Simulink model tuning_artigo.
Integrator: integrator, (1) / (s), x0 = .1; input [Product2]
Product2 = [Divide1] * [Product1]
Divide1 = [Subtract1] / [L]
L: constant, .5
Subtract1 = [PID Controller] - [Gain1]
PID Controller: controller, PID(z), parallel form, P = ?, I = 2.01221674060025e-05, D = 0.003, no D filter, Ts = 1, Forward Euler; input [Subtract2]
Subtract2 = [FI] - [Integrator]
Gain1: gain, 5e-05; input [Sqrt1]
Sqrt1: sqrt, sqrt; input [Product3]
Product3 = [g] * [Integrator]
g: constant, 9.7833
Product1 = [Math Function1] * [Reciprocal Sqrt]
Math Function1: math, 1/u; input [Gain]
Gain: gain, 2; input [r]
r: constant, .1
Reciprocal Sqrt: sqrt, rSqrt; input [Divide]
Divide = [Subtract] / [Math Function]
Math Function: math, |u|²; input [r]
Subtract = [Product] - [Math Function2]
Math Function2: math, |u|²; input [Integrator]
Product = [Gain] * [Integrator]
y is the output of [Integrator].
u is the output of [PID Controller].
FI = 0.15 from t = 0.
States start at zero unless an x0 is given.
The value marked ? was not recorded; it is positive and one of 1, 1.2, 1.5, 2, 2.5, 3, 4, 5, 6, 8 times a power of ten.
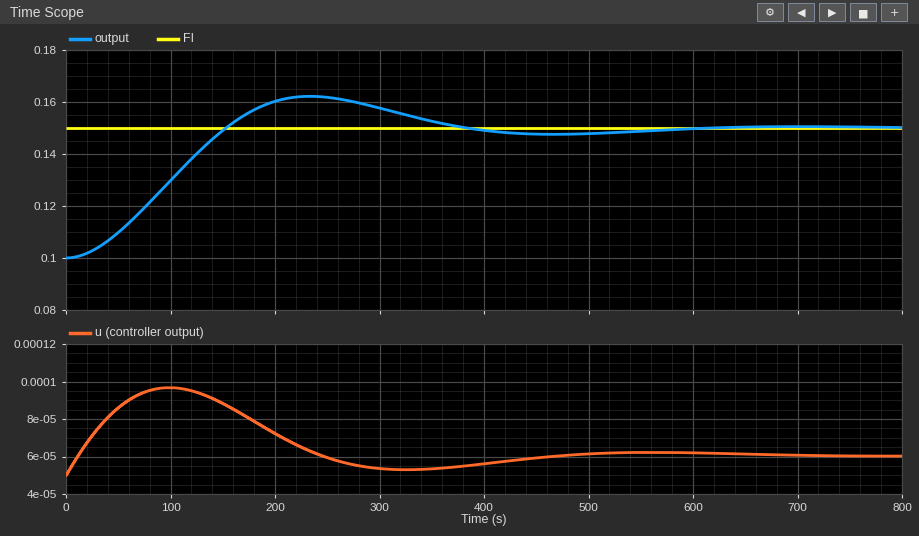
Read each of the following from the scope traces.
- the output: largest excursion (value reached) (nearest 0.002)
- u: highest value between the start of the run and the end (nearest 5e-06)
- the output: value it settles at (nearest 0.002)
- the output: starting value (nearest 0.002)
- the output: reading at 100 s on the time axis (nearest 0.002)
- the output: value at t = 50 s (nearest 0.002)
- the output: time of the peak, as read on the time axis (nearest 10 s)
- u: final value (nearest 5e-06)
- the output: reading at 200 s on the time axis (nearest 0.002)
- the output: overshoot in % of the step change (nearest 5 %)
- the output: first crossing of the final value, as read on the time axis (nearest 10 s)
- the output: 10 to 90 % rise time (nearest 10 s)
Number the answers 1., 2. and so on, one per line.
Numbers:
1. 0.162
2. 0.000095
3. 0.150
4. 0.100
5. 0.130
6. 0.110
7. 230 s
8. 0.000060
9. 0.160
10. 25 %
11. 150 s
12. 100 s
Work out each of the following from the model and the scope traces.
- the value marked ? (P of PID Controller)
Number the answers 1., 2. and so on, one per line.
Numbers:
1. 0.001
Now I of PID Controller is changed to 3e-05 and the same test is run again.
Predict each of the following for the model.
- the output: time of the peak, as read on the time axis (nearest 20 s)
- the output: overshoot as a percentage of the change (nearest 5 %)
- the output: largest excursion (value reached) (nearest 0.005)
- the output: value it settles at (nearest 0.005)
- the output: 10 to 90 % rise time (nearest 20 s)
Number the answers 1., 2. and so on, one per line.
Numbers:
1. 180 s
2. 35 %
3. 0.165
4. 0.150
5. 80 s
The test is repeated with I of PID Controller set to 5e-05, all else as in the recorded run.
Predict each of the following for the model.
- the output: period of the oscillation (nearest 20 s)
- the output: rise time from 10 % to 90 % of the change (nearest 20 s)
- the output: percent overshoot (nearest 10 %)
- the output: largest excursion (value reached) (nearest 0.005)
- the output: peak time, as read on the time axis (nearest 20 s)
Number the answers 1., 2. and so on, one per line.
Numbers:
1. 280 s
2. 60 s
3. 50 %
4. 0.175
5. 140 s
